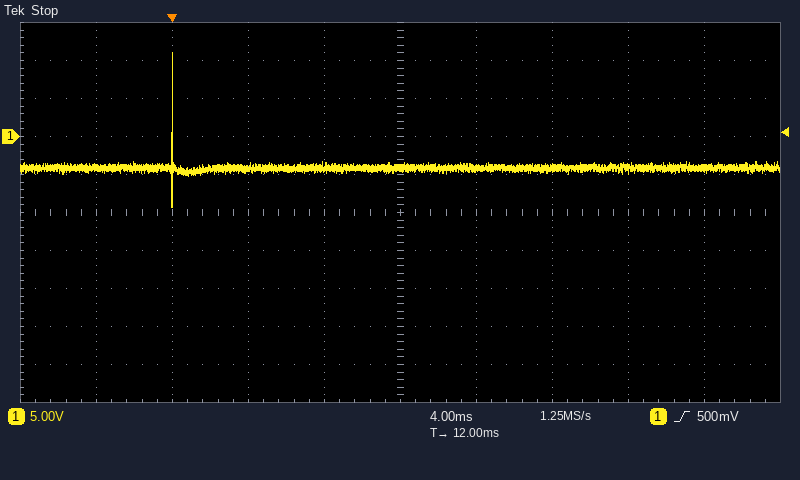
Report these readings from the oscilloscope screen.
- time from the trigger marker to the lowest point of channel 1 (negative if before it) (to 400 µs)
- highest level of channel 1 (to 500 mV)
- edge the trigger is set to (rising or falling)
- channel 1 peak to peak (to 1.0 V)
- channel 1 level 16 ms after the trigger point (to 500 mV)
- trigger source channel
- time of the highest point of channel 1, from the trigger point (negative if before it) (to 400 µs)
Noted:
0.0 ms
11.0 V
rising
20.0 V
-4.0 V
channel 1
0.0 ms
